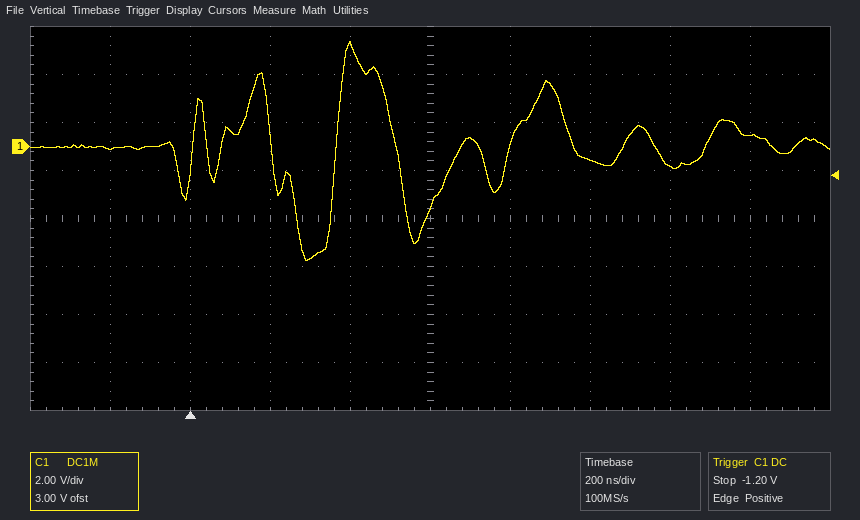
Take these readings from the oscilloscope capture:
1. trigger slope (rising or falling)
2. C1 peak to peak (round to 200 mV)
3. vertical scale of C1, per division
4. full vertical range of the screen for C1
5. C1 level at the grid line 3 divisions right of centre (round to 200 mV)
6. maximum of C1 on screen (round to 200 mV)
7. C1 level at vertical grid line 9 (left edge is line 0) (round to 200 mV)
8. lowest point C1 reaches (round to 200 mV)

rising
9.2 V
2 V
16 V
-800 mV
4.4 V
400 mV
-4.8 V
